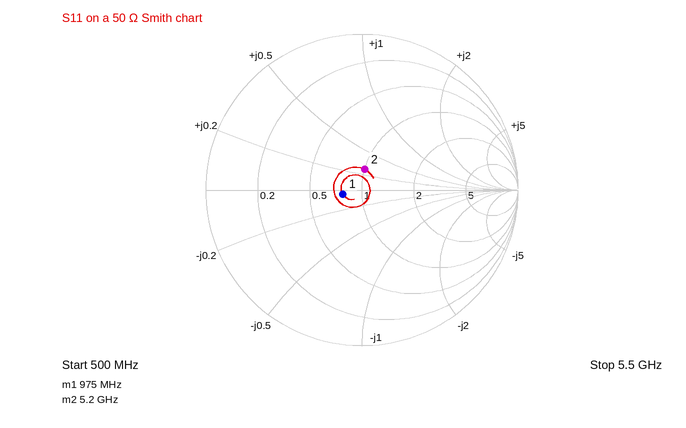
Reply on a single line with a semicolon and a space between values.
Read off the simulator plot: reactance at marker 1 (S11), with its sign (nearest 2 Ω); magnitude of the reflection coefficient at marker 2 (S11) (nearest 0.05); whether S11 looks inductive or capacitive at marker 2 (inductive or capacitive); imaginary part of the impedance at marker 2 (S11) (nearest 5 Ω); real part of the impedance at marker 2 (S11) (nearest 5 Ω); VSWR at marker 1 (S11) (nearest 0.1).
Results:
-2 Ω; 0.15; inductive; +15 Ω; 50 Ω; 1.3
